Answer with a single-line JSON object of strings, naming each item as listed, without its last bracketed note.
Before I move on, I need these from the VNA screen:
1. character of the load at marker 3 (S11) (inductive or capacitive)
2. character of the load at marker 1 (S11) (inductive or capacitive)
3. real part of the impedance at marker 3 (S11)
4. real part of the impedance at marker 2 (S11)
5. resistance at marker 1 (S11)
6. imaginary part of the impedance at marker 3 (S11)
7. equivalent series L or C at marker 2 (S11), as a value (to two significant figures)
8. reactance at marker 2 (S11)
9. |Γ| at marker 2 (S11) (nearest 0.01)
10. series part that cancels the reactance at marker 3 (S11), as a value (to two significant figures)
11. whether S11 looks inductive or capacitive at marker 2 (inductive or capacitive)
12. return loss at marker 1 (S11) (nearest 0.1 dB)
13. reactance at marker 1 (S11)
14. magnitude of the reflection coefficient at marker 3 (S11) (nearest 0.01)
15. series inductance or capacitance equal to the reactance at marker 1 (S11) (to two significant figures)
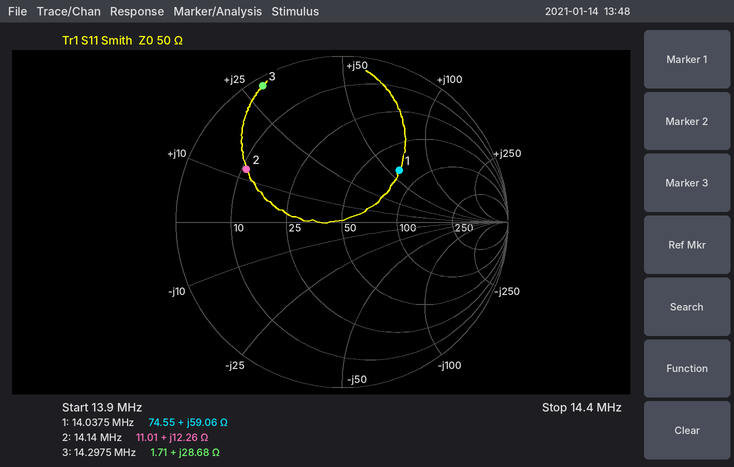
{"character of the load at marker 3 (S11)": "inductive", "character of the load at marker 1 (S11)": "inductive", "real part of the impedance at marker 3": "1.71 Ω", "real part of the impedance at marker 2": "11.01 Ω", "resistance at marker 1": "74.55 Ω", "imaginary part of the impedance at marker 3": "+28.68 Ω", "equivalent series L or C at marker 2 (S11), as a value": "140 nH", "reactance at marker 2": "+12.26 Ω", "|Γ| at marker 2 (S11)": "0.66", "series part that cancels the reactance at marker 3 (S11), as a value": "390 pF", "whether S11 looks inductive or capacitive at marker 2": "inductive", "return loss at marker 1 (S11)": "6.7 dB", "reactance at marker 1": "+59.06 Ω", "magnitude of the reflection coefficient at marker 3 (S11)": "0.95", "series inductance or capacitance equal to the reactance at marker 1 (S11)": "670 nH"}
